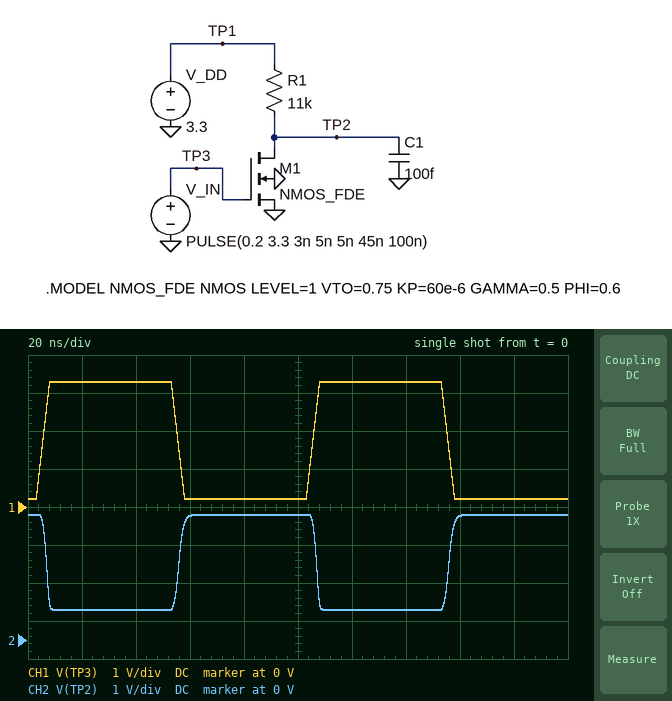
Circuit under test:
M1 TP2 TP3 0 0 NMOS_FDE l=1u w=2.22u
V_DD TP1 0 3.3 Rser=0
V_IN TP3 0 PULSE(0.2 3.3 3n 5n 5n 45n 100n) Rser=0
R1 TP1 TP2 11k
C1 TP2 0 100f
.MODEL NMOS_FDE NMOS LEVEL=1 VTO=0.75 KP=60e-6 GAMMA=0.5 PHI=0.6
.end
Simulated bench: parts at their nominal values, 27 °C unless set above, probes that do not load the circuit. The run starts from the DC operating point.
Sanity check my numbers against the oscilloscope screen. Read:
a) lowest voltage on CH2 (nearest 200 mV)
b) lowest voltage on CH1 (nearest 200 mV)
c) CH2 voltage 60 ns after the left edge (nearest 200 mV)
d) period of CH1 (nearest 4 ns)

800 mV
200 mV
3.2 V
100 ns
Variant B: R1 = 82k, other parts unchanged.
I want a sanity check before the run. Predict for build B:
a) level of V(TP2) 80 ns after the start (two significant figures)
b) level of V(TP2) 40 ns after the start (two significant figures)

3.1 V
120 mV
